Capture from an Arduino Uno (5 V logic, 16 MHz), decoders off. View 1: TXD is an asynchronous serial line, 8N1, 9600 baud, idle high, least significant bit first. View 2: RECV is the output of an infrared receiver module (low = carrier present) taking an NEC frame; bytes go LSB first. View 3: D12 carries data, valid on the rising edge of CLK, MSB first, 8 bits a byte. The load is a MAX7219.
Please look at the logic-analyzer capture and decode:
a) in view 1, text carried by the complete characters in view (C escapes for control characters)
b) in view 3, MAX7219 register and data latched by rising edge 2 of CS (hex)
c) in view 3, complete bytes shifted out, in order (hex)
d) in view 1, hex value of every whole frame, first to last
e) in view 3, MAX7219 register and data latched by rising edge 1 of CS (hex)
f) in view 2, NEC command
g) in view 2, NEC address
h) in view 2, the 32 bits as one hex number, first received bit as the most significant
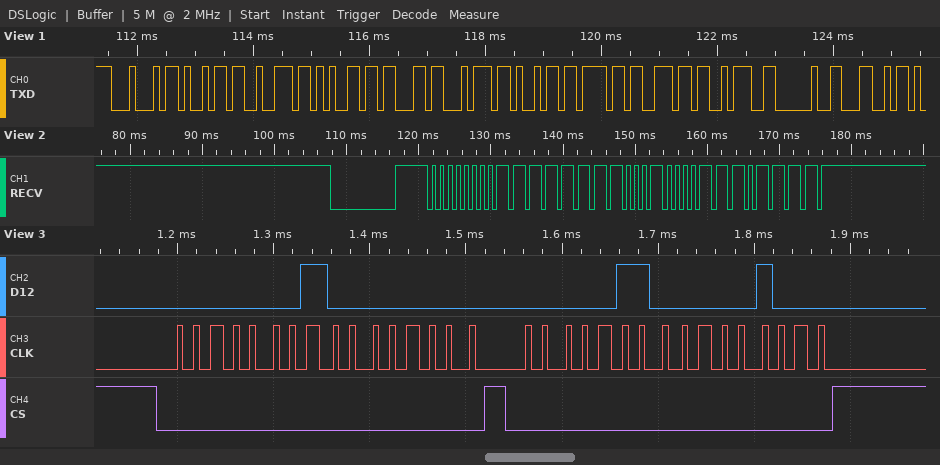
"Direction: L"
register 0x6, data 0x08
01 00 06 08
44 69 72 65 63 74 69 6F 6E 3A 20 4C
register 0x1, data 0x00
0x08
0x00
0x00FF10EF
